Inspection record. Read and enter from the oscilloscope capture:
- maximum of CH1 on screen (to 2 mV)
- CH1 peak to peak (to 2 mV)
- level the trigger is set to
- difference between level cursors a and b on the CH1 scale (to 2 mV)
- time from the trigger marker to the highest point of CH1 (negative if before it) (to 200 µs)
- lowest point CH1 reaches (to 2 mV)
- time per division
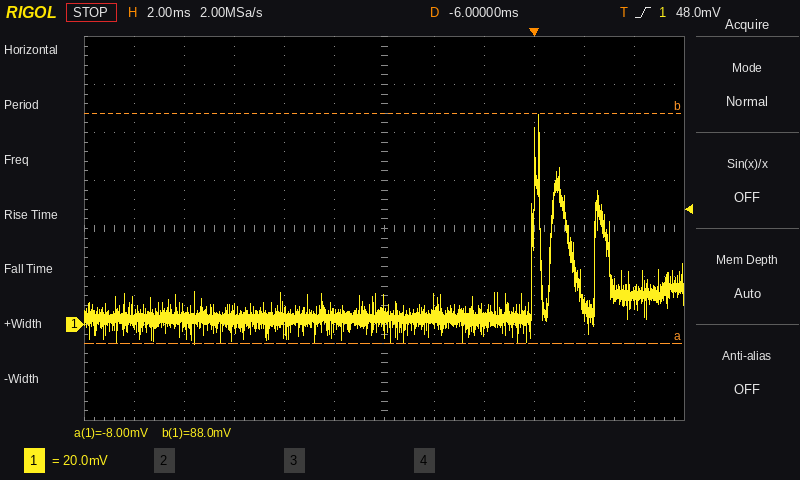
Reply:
88 mV
96 mV
48.0 mV
96 mV
+200 µs
-8 mV
2 ms
